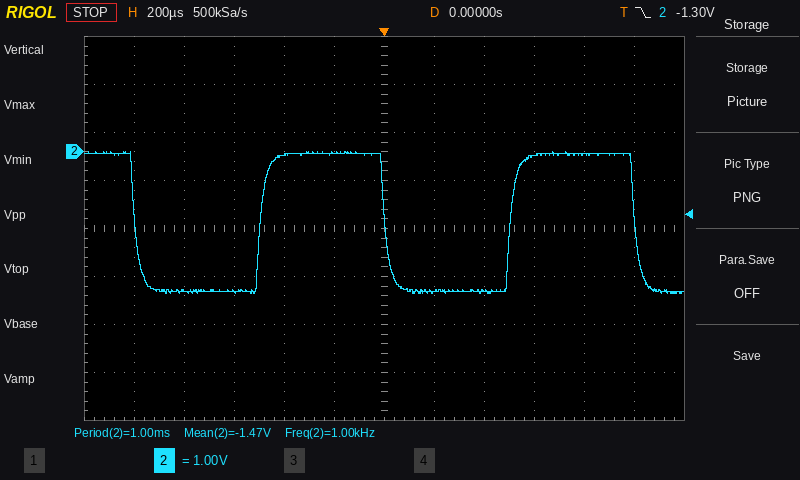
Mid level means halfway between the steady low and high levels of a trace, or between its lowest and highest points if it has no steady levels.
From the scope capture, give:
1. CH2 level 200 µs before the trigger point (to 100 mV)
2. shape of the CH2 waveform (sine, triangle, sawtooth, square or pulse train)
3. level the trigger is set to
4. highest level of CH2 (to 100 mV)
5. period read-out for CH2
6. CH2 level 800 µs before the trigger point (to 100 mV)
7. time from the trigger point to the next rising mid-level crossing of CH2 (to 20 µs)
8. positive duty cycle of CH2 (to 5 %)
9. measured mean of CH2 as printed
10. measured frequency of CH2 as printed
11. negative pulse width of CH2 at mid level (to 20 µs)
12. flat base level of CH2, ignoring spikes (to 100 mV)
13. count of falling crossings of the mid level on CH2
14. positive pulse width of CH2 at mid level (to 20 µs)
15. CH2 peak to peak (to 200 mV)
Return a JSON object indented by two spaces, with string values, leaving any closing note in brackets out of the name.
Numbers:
{
  "CH2 level 200 µs before the trigger point": "0.0 V",
  "shape of the CH2 waveform": "square",
  "level the trigger is set to": "-1.30 V",
  "highest level of CH2": "0.0 V",
  "period read-out for CH2": "1.00 ms",
  "CH2 level 800 µs before the trigger point": "-2.9 V",
  "time from the trigger point to the next rising mid-level crossing of CH2": "500 µs",
  "positive duty cycle of CH2": "50 %",
  "measured mean of CH2 as printed": "-1.47 V",
  "measured frequency of CH2 as printed": "1.00 kHz",
  "negative pulse width of CH2 at mid level": "500 µs",
  "flat base level of CH2, ignoring spikes": "-2.9 V",
  "count of falling crossings of the mid level on CH2": "3",
  "positive pulse width of CH2 at mid level": "500 µs",
  "CH2 peak to peak": "3.0 V"
}
